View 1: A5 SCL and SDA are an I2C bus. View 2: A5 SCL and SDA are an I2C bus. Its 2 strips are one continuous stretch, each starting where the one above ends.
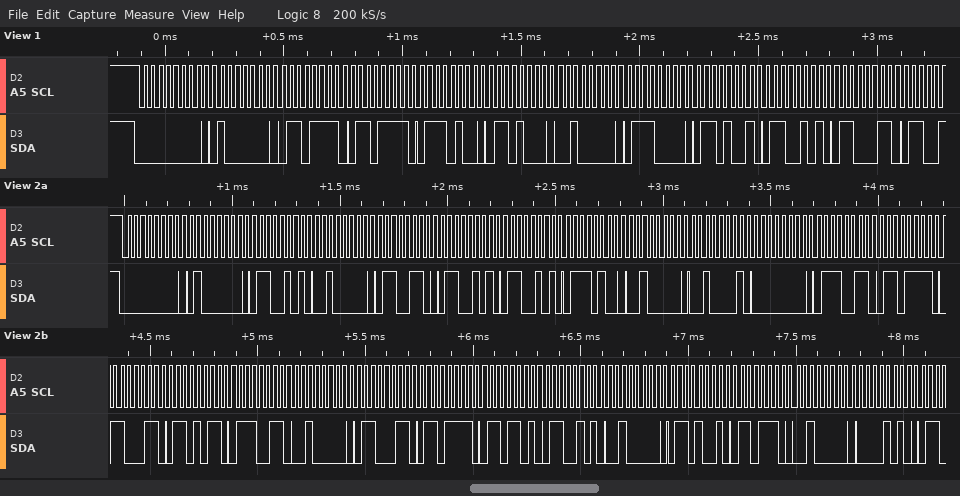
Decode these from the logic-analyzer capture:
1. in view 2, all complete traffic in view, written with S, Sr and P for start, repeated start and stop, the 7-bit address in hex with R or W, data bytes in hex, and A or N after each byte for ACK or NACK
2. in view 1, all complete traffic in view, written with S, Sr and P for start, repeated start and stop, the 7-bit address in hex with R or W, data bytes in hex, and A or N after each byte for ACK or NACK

S 00W A 40 A 65 A 20 A 66 A 65 A 65 A 74 A 20 A 21 A 00 A 73 A 6F A 63 A 6B A 73 A 20 A 63 A 6F A 6D A 65 A 20 A 69 A 6E A 20 A 0A A
S 00W A 40 A 6F A 6F A 74 A 68 A 20 A 70 A 69 A 65 A 63 A
